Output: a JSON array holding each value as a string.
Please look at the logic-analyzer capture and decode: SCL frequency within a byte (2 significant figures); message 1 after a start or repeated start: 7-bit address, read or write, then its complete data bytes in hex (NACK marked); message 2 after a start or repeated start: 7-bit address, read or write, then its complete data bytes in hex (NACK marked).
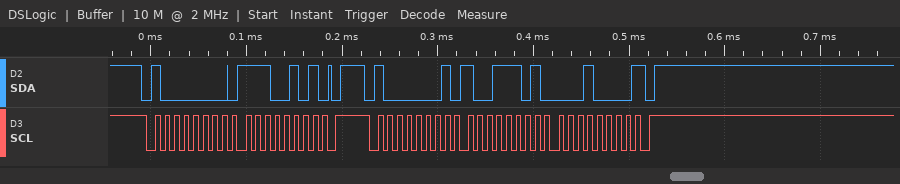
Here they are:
["100 kHz", "0x40 write: E5", "0x40 read: 9D 10 NACK"]
